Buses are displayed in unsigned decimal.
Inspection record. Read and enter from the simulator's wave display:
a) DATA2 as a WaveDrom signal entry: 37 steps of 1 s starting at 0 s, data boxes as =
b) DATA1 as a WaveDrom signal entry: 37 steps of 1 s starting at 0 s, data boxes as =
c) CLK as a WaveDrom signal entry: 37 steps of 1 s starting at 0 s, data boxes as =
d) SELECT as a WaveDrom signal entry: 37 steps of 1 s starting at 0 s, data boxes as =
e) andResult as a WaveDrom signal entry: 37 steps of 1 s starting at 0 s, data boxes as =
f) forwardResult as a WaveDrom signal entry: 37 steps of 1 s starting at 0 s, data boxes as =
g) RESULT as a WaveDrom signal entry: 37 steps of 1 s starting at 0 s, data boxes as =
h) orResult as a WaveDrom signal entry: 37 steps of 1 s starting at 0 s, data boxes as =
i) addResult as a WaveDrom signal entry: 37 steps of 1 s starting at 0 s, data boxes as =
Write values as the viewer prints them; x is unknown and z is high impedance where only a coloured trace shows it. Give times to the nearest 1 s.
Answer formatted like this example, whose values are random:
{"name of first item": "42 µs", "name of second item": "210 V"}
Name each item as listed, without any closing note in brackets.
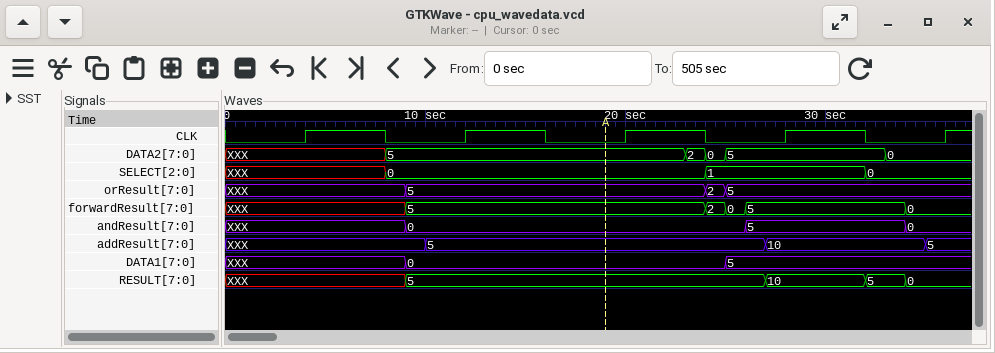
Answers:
{"DATA2 as a WaveDrom signal entry: 37 steps of 1 s starting at 0 s, data boxes as =": "{name: 'DATA2', wave: 'x.......=..............===.......=...', data: '5 2 0 5 0'}", "DATA1 as a WaveDrom signal entry: 37 steps of 1 s starting at 0 s, data boxes as =": "{name: 'DATA1', wave: 'x........=...............=...........', data: '0 5'}", "CLK as a WaveDrom signal entry: 37 steps of 1 s starting at 0 s, data boxes as =": "{name: 'CLK', wave: '0...1...0...1...0...1...0...1...0...1'}", "SELECT as a WaveDrom signal entry: 37 steps of 1 s starting at 0 s, data boxes as =": "{name: 'SELECT', wave: 'x.......=...............=.......=....', data: '0 1 0'}", "andResult as a WaveDrom signal entry: 37 steps of 1 s starting at 0 s, data boxes as =": "{name: 'andResult', wave: 'x........=................=.......=..', data: '0 5 0'}", "forwardResult as a WaveDrom signal entry: 37 steps of 1 s starting at 0 s, data boxes as =": "{name: 'forwardResult', wave: 'x........=..............===.......=..', data: '5 2 0 5 0'}", "RESULT as a WaveDrom signal entry: 37 steps of 1 s starting at 0 s, data boxes as =": "{name: 'RESULT', wave: 'x........=.................=....=.=..', data: '5 10 5 0'}", "orResult as a WaveDrom signal entry: 37 steps of 1 s starting at 0 s, data boxes as =": "{name: 'orResult', wave: 'x........=..............==...........', data: '5 2 5'}", "addResult as a WaveDrom signal entry: 37 steps of 1 s starting at 0 s, data boxes as =": "{name: 'addResult', wave: 'x.........=................=.......=.', data: '5 10 5'}"}
